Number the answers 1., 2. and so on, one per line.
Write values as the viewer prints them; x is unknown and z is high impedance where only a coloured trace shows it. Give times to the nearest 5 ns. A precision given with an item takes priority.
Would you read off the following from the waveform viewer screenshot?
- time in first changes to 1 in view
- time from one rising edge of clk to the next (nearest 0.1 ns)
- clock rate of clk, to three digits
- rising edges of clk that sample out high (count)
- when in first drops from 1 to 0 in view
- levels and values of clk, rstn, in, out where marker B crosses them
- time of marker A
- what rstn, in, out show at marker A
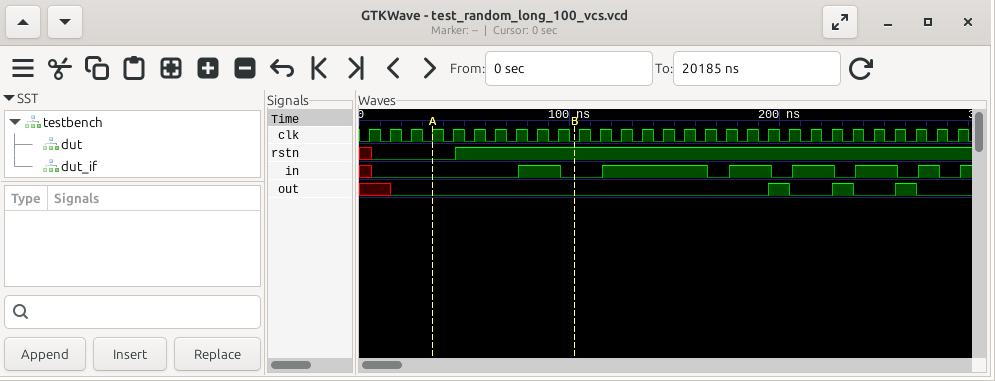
1. 75 ns
2. 10 ns
3. 100 MHz
4. 3
5. 95 ns
6. clk=0, rstn=1, in=0, out=0
7. 35 ns
8. rstn=0, in=0, out=0
